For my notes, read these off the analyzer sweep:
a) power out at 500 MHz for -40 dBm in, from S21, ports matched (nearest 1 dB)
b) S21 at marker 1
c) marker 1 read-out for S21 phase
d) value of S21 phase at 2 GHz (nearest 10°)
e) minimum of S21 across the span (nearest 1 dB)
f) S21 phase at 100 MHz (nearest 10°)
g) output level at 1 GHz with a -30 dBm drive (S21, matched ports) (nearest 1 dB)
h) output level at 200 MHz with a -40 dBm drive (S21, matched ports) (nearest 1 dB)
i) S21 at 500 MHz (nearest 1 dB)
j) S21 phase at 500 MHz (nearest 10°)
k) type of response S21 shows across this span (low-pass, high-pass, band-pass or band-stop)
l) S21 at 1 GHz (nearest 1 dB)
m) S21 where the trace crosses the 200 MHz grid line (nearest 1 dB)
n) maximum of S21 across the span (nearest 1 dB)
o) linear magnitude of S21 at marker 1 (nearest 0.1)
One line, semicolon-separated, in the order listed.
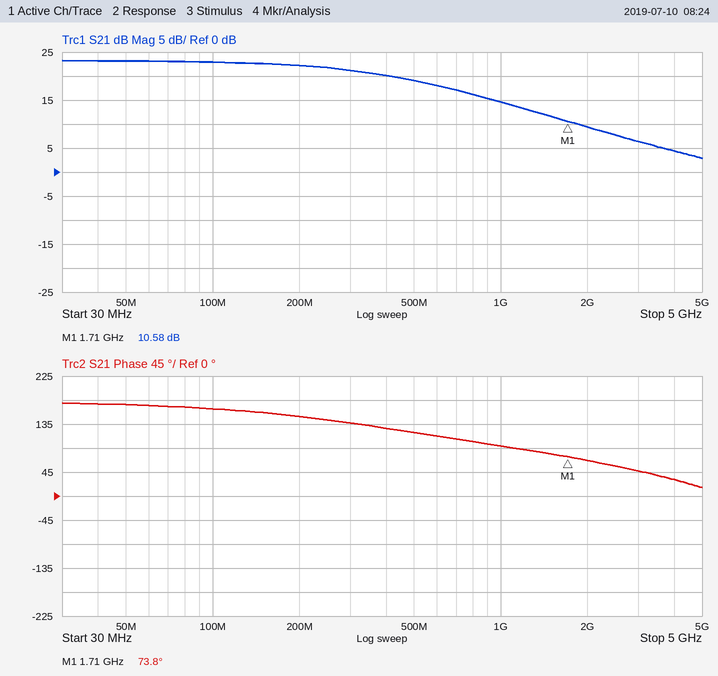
-21 dBm; 10.58 dB; 73.8°; 70°; 3 dB; 160°; -15 dBm; -18 dBm; 19 dB; 120°; low-pass; 15 dB; 22 dB; 23 dB; 3.4
